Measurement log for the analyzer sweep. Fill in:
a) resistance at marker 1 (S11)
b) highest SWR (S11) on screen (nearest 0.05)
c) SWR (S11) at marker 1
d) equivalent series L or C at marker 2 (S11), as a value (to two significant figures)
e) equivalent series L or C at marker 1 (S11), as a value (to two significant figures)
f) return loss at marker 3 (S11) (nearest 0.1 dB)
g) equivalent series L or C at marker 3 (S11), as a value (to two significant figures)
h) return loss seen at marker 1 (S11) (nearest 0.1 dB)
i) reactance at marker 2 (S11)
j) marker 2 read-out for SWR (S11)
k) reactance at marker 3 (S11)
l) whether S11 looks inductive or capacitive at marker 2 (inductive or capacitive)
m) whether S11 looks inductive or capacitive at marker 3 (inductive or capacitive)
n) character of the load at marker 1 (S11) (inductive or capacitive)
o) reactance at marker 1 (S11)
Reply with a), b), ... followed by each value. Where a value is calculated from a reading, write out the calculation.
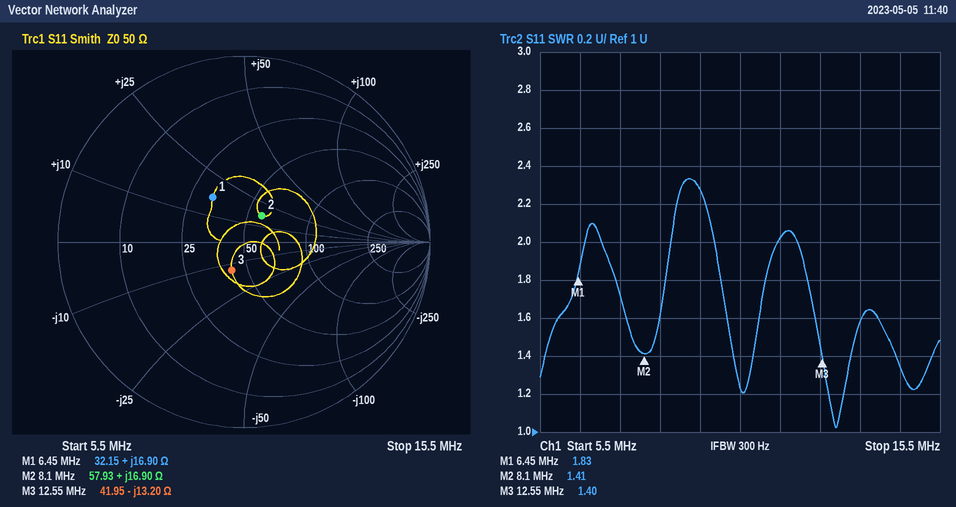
a) 32.15 Ω
b) 2.35
c) 1.83
d) L = 16.9 Ω/(2π × 8.1 MHz) ≈ 332 nH, so 330 nH to two significant figures
e) L = 16.9 Ω/(2π × 6.45 MHz) ≈ 417 nH, so 420 nH to two significant figures
f) 15.6 dB
g) C = 1/(2π × 12.55 MHz × 13.2 Ω) ≈ 961 pF, so 960 pF to two significant figures
h) 10.7 dB
i) +16.90 Ω
j) 1.41
k) -13.20 Ω
l) inductive
m) capacitive
n) inductive
o) +16.90 Ω
